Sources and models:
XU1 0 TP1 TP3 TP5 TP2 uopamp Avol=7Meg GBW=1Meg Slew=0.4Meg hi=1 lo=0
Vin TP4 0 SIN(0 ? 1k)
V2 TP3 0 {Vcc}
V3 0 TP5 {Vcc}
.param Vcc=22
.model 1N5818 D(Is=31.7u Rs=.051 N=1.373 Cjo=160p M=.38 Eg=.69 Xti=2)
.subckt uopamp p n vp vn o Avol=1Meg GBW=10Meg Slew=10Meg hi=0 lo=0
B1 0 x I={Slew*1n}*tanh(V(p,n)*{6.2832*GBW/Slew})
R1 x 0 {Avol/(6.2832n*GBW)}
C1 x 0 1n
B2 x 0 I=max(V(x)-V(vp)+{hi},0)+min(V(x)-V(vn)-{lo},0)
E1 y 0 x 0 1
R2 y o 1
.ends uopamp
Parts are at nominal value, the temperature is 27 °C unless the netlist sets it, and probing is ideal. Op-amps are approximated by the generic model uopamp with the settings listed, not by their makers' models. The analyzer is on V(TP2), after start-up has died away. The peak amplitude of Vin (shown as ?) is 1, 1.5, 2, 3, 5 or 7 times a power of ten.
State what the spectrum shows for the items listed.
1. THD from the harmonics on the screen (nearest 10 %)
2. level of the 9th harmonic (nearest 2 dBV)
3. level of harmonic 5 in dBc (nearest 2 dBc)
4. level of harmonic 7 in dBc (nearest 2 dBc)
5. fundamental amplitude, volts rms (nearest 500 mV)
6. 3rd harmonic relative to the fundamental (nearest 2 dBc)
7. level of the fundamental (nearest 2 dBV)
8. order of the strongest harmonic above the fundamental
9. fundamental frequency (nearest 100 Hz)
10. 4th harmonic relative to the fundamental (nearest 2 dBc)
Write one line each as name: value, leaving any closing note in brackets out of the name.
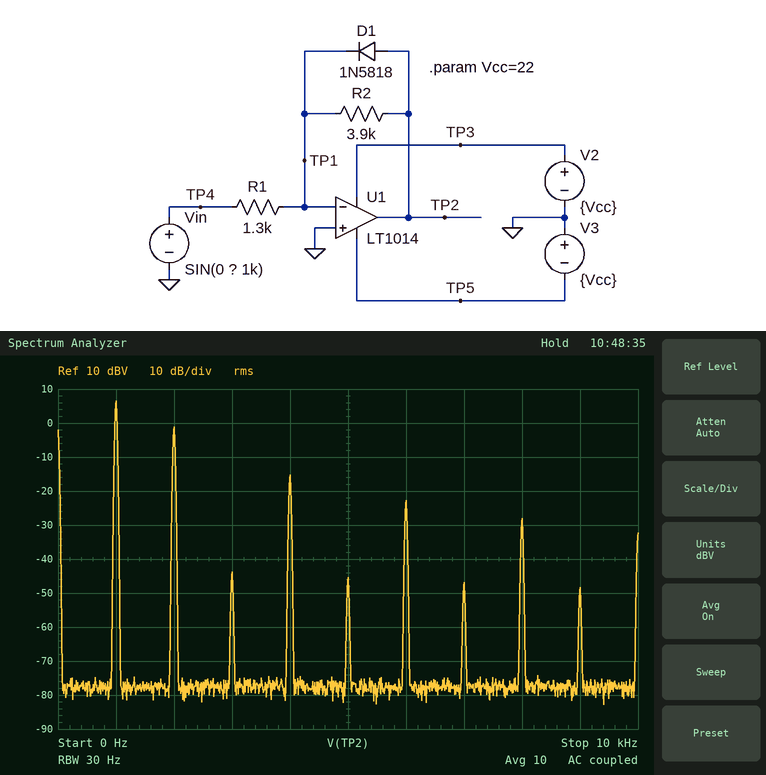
THD from the harmonics on the screen: 40 %
level of the 9th harmonic: -48 dBV
level of harmonic 5 in dBc: -52 dBc
level of harmonic 7 in dBc: -54 dBc
fundamental amplitude, volts rms: 2.0 V
3rd harmonic relative to the fundamental: -50 dBc
level of the fundamental: 6 dBV
order of the strongest harmonic above the fundamental: 2
fundamental frequency: 1.0 kHz
4th harmonic relative to the fundamental: -22 dBc
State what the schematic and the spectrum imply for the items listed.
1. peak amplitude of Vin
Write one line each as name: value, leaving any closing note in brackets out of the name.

peak amplitude of Vin: 2 V
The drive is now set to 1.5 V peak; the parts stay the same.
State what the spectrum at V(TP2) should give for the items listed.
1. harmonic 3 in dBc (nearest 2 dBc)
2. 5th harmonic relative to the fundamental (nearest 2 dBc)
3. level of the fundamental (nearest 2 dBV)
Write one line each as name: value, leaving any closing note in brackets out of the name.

harmonic 3 in dBc: -46 dBc
5th harmonic relative to the fundamental: -48 dBc
level of the fundamental: 4 dBV
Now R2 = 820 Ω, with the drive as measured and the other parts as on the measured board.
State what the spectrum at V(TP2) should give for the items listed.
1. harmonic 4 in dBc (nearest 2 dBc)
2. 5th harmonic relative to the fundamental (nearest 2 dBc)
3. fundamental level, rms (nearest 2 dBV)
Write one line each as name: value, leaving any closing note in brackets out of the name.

harmonic 4 in dBc: -24 dBc
5th harmonic relative to the fundamental: -46 dBc
fundamental level, rms: -6 dBV
